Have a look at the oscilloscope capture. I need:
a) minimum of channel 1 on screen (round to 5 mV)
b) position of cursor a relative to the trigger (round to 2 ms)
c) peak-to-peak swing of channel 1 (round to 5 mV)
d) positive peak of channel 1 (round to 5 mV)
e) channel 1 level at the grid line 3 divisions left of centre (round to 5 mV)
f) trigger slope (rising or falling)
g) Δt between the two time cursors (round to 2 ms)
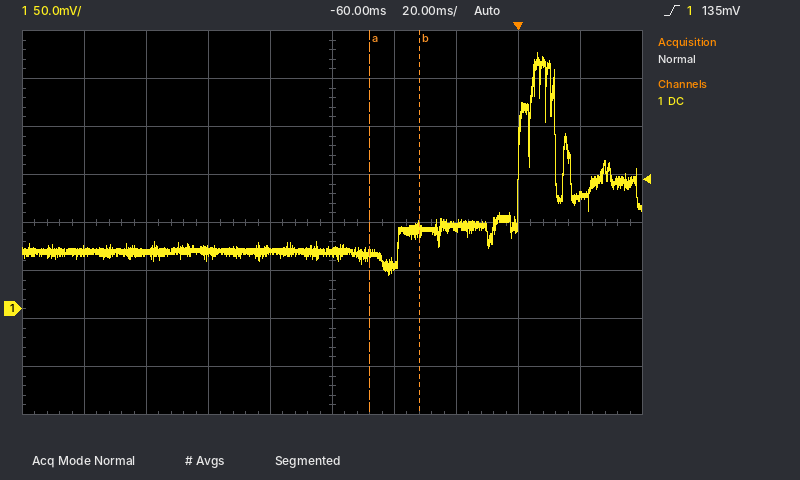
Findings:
35 mV
-48 ms
230 mV
265 mV
60 mV
rising
16 ms
